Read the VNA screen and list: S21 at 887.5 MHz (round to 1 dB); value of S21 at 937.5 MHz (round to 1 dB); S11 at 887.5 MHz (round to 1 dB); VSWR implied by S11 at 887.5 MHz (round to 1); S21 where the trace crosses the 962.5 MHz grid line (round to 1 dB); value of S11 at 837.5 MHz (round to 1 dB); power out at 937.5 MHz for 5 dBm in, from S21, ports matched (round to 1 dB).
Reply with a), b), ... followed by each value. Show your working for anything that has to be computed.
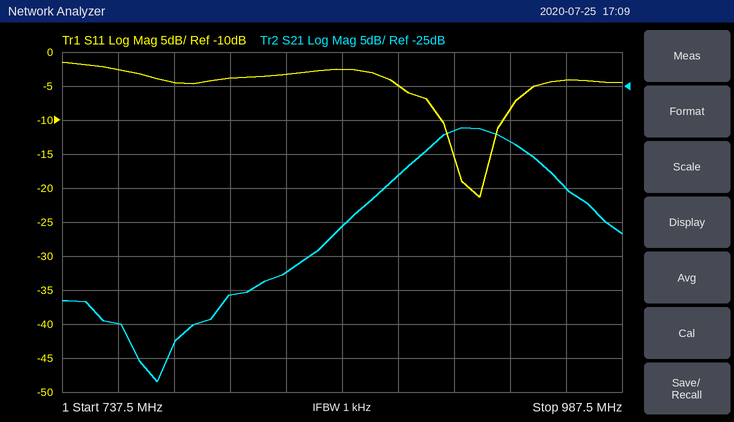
a) -38 dB
b) -33 dB
c) -5 dB
d) |Γ| = 10^(-5/20) = 0.5623; VSWR = (1 + 0.5623)/(1 − 0.5623) ≈ 4
e) -40 dB
f) -3 dB
g) 5 dBm + (-33 dB) = -28 dBm
